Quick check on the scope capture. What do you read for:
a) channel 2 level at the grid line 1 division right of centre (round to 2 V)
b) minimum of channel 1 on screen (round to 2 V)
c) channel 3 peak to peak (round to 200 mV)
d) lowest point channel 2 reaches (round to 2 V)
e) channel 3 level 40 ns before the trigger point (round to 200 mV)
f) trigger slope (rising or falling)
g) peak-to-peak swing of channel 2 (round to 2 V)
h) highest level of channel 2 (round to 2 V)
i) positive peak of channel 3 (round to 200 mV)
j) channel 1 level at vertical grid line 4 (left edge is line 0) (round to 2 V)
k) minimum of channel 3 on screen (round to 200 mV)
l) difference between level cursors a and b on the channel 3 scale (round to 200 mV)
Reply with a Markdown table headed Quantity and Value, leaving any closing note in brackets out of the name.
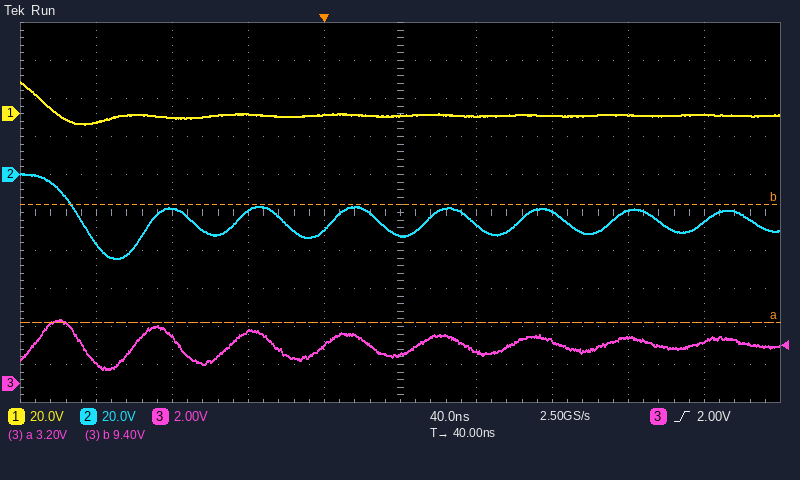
| Quantity | Value |
|---|---|
| channel 2 level at the grid line 1 division right of centre | -26 V |
| minimum of channel 1 on screen | -6 V |
| channel 3 peak to peak | 2.6 V |
| lowest point channel 2 reaches | -44 V |
| channel 3 level 40 ns before the trigger point | 2.8 V |
| trigger slope | rising |
| peak-to-peak swing of channel 2 | 44 V |
| highest level of channel 2 | 0 V |
| positive peak of channel 3 | 3.4 V |
| channel 1 level at vertical grid line 4 (left edge is line 0) | 0 V |
| minimum of channel 3 on screen | 800 mV |
| difference between level cursors a and b on the channel 3 scale | 6.2 V |
